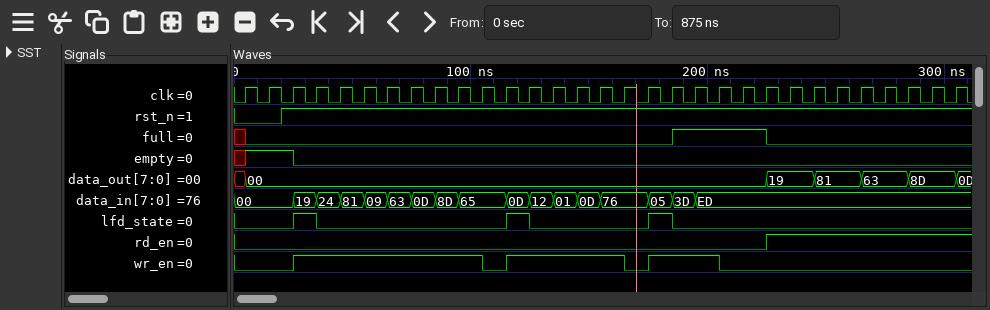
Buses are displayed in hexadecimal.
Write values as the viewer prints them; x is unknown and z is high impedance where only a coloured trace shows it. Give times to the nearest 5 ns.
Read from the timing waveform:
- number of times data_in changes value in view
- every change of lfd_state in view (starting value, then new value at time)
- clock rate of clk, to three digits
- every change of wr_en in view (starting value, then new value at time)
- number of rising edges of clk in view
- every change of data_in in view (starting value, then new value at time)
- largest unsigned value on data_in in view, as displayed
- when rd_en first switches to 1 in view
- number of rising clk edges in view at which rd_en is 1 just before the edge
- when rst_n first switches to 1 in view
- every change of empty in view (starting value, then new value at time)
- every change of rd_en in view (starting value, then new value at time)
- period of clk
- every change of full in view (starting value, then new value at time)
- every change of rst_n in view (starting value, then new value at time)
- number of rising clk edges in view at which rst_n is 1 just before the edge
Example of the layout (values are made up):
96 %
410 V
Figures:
16
0, 1 at 25 ns, 0 at 35 ns, 1 at 115 ns, 0 at 125 ns, 1 at 175 ns, 0 at 185 ns
100 MHz
0, 1 at 25 ns, 0 at 105 ns, 1 at 115 ns, 0 at 165 ns, 1 at 175 ns, 0 at 205 ns
31
00, 19 at 25 ns, 24 at 35 ns, 81 at 45 ns, 09 at 55 ns, 63 at 65 ns, 0D at 75 ns, 8D at 85 ns, 65 at 95 ns, 0D at 115 ns, 12 at 125 ns, 01 at 135 ns, 0D at 145 ns, 76 at 155 ns, 05 at 175 ns, 3D at 185 ns, ED at 195 ns
ED
225 ns
8
20 ns
x, 1 at 5 ns, 0 at 25 ns
0, 1 at 225 ns
10 ns
x, 0 at 5 ns, 1 at 185 ns, 0 at 225 ns
0, 1 at 20 ns
29
